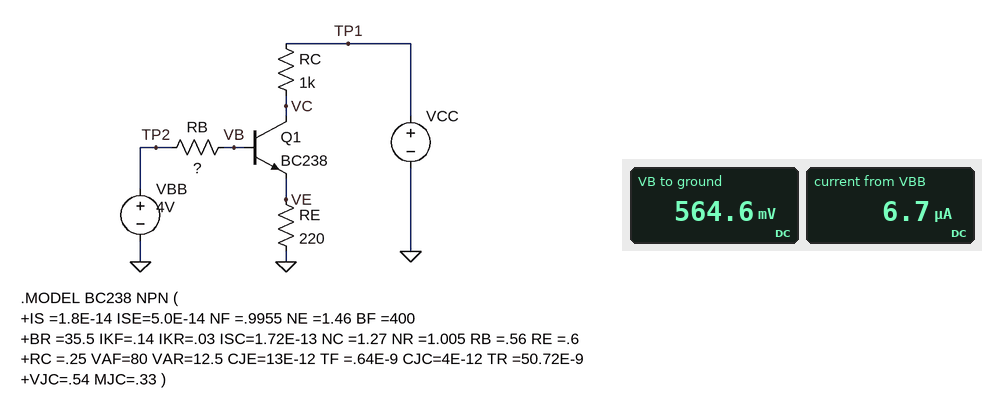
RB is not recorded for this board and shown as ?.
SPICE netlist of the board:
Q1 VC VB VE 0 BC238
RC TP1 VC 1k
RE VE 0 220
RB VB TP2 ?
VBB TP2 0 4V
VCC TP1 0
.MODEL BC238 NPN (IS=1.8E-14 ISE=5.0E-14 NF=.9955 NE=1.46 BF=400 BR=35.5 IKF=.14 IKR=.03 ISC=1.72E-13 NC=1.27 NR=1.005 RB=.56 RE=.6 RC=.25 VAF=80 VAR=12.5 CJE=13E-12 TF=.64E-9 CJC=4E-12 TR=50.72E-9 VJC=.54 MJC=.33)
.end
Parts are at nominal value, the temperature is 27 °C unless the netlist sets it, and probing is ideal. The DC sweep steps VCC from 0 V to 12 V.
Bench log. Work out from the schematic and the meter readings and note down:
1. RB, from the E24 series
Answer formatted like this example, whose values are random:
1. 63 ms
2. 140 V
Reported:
1. 510 kΩ
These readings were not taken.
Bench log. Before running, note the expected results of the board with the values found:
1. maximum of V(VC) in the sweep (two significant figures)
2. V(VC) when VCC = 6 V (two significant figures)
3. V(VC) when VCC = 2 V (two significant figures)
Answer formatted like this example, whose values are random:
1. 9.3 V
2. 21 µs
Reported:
1. 10 V
2. 4.3 V
3. 500 mV
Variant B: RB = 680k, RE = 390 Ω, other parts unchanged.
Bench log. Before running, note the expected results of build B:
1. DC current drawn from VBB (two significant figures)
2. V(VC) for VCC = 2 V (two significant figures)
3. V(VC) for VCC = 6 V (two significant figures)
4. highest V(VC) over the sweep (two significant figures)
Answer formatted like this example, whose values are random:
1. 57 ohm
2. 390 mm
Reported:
1. 5.1 µA
2. 850 mV
3. 4.8 V
4. 11 V
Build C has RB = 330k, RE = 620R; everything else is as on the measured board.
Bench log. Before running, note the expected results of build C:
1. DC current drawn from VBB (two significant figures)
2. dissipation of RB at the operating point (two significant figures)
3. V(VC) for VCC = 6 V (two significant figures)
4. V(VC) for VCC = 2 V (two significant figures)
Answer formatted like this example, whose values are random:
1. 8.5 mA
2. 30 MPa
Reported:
1. 10 µA
2. 35 µW
3. 4.1 V
4. 830 mV
